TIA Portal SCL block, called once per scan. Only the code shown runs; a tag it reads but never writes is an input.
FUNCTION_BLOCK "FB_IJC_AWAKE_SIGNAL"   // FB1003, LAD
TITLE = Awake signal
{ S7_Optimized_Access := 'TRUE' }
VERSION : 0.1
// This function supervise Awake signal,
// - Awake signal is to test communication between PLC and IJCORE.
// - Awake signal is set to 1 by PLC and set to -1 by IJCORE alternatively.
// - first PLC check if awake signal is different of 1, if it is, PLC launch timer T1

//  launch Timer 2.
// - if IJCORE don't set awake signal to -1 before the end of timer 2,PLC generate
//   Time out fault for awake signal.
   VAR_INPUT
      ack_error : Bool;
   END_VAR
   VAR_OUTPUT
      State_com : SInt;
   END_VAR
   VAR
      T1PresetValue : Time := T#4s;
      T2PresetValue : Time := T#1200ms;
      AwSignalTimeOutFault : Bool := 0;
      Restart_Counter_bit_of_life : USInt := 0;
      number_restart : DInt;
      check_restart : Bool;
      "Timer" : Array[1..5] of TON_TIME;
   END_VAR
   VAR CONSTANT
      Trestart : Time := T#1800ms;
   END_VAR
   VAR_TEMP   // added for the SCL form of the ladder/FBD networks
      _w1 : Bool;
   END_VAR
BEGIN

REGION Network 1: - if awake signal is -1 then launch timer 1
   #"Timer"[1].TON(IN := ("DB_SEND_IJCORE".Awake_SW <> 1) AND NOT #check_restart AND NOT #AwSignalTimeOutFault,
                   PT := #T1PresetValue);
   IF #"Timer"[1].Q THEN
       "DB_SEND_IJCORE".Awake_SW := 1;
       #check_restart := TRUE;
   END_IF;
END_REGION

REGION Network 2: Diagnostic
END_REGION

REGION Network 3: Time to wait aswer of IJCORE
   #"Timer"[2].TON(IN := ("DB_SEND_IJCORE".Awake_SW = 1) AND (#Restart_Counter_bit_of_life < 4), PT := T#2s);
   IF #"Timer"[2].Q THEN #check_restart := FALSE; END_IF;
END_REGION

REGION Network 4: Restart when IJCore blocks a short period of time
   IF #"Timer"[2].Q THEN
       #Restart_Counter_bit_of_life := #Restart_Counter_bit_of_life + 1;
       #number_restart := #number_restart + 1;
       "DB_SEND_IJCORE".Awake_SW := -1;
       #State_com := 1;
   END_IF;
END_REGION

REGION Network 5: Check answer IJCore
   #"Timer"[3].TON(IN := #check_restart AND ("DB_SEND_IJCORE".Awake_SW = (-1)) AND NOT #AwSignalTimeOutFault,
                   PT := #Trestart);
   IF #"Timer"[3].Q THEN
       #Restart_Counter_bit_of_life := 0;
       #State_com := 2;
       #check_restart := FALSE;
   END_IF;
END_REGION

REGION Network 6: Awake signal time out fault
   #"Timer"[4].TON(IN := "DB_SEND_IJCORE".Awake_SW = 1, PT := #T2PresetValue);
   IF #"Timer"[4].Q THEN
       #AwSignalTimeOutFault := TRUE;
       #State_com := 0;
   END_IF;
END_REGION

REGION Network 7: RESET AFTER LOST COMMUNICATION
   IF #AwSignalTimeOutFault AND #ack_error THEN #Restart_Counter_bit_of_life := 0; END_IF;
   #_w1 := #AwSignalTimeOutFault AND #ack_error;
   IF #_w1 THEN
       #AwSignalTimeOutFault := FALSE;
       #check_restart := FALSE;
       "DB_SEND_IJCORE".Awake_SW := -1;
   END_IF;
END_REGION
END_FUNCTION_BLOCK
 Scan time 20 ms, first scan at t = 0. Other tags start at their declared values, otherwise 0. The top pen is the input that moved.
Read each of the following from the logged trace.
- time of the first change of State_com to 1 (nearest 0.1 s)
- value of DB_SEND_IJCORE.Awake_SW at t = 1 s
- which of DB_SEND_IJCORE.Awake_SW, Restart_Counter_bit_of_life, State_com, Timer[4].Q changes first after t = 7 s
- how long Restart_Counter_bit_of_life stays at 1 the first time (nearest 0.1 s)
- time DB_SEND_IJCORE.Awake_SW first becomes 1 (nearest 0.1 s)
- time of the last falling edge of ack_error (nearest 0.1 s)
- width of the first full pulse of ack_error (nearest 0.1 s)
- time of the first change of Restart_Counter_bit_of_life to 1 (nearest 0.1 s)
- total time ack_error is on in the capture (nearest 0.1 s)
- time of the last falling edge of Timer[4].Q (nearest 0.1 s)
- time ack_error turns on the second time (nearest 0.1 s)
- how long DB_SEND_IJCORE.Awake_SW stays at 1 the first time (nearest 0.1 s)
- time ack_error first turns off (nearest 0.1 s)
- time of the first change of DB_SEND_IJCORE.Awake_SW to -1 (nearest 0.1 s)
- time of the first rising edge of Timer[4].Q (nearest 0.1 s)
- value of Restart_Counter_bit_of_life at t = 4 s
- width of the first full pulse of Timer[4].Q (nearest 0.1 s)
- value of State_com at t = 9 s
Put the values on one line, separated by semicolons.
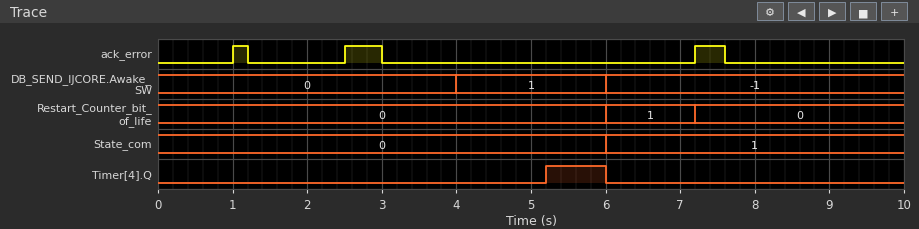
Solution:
6.0 s; 0; Restart_Counter_bit_of_life; 1.2 s; 4.0 s; 7.6 s; 0.2 s; 6.0 s; 1.1 s; 6.0 s; 2.5 s; 2.0 s; 1.2 s; 6.0 s; 5.2 s; 0; 0.8 s; 1
